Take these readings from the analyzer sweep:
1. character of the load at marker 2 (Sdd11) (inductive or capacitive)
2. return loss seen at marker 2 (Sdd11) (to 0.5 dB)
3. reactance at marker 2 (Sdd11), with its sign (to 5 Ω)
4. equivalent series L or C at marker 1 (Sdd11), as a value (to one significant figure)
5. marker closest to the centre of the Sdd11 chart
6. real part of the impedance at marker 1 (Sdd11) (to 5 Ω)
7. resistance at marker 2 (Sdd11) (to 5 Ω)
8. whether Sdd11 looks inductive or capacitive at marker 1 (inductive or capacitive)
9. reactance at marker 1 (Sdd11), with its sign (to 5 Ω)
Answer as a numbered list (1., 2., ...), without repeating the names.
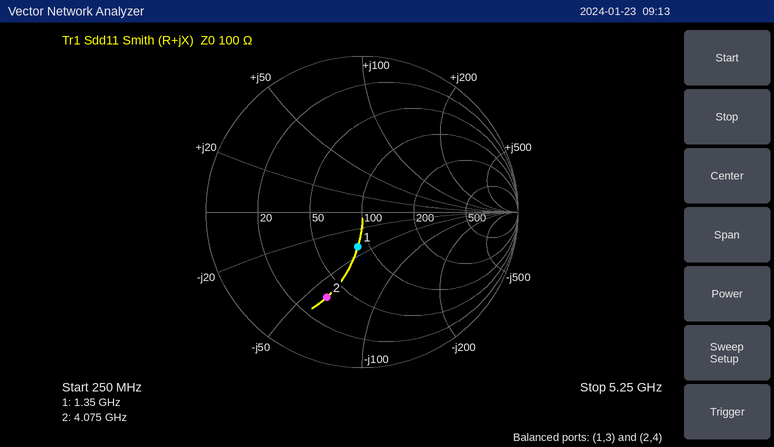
1. capacitive
2. 4.5 dB
3. -60 Ω
4. 3 pF
5. marker 1
6. 85 Ω
7. 35 Ω
8. capacitive
9. -40 Ω
